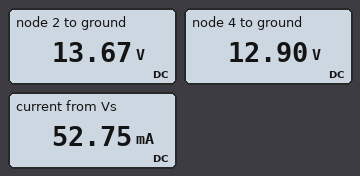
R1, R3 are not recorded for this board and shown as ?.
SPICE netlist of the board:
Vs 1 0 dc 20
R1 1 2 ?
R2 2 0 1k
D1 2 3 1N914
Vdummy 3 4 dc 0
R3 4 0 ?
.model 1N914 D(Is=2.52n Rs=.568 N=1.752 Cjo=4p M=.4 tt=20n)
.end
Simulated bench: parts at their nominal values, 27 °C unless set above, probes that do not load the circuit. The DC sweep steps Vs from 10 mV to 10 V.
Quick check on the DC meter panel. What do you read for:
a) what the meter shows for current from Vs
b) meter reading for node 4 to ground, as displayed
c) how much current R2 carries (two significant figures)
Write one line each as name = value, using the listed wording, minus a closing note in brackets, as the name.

what the meter shows for current from Vs = 52.75 mA
meter reading for node 4 to ground, as displayed = 12.90 V
how much current R2 carries = 14 mA
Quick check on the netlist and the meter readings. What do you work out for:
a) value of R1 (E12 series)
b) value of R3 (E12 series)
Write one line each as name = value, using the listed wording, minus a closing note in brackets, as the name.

value of R1 = 120 Ω
value of R3 = 330 Ω
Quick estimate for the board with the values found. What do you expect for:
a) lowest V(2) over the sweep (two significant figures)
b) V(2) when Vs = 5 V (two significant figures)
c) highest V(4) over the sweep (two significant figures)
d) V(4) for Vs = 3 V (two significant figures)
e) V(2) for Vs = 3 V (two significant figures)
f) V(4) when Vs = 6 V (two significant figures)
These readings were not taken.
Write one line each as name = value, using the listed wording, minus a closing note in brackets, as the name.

lowest V(2) over the sweep = 8.9 mV
V(2) when Vs = 5 V = 3.5 V
highest V(4) over the sweep = 6.2 V
V(4) for Vs = 3 V = 1.5 V
V(2) for Vs = 3 V = 2.2 V
V(4) when Vs = 6 V = 3.5 V
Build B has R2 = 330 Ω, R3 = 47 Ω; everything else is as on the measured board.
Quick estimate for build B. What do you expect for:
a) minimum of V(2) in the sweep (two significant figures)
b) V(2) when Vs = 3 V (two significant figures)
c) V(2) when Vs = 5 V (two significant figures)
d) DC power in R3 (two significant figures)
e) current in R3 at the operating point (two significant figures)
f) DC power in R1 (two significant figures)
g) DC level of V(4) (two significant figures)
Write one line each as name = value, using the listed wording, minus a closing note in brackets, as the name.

minimum of V(2) in the sweep = 7.3 mV
V(2) when Vs = 3 V = 1.2 V
V(2) when Vs = 5 V = 1.8 V
DC power in R3 = 490 mW
current in R3 at the operating point = 100 mA
DC power in R1 = 1.7 W
DC level of V(4) = 4.8 V
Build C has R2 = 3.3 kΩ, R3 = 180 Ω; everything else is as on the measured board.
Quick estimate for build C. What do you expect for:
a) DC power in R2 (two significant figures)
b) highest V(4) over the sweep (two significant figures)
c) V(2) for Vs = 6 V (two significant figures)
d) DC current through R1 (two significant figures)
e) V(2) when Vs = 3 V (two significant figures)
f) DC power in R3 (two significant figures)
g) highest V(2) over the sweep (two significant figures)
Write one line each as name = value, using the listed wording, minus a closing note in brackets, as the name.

DC power in R2 = 44 mW
highest V(4) over the sweep = 5.4 V
V(2) for Vs = 6 V = 3.8 V
DC current through R1 = 66 mA
V(2) when Vs = 3 V = 2.0 V
DC power in R3 = 700 mW
highest V(2) over the sweep = 6.2 V
